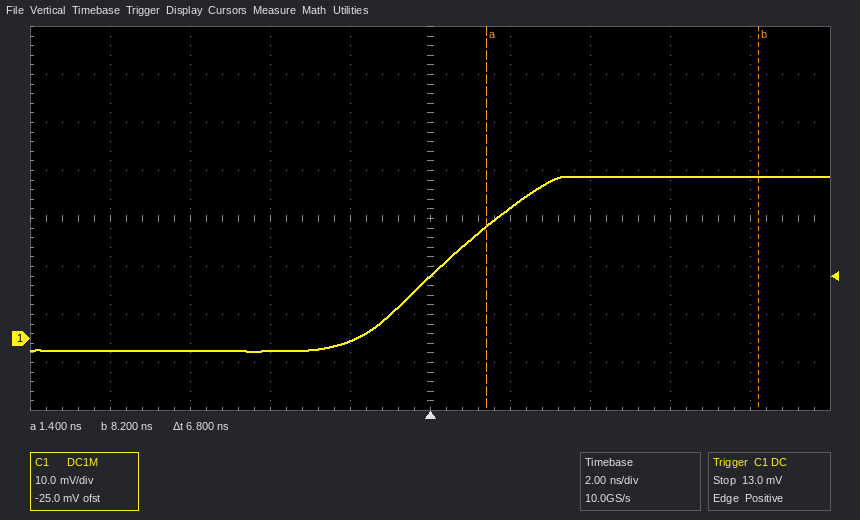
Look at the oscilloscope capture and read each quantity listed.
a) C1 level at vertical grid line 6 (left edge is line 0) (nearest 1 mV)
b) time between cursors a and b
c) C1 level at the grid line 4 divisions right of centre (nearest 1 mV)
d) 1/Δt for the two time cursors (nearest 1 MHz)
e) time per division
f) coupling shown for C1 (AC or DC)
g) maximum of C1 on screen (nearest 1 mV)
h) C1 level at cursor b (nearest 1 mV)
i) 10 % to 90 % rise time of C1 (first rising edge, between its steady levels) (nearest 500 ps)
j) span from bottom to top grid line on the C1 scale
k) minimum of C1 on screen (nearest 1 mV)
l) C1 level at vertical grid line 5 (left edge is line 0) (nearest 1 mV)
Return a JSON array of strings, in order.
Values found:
["27 mV", "6.8 ns", "34 mV", "147 MHz", "2 ns", "DC", "34 mV", "34 mV", "4.0 ns", "80 mV", "-3 mV", "13 mV"]
